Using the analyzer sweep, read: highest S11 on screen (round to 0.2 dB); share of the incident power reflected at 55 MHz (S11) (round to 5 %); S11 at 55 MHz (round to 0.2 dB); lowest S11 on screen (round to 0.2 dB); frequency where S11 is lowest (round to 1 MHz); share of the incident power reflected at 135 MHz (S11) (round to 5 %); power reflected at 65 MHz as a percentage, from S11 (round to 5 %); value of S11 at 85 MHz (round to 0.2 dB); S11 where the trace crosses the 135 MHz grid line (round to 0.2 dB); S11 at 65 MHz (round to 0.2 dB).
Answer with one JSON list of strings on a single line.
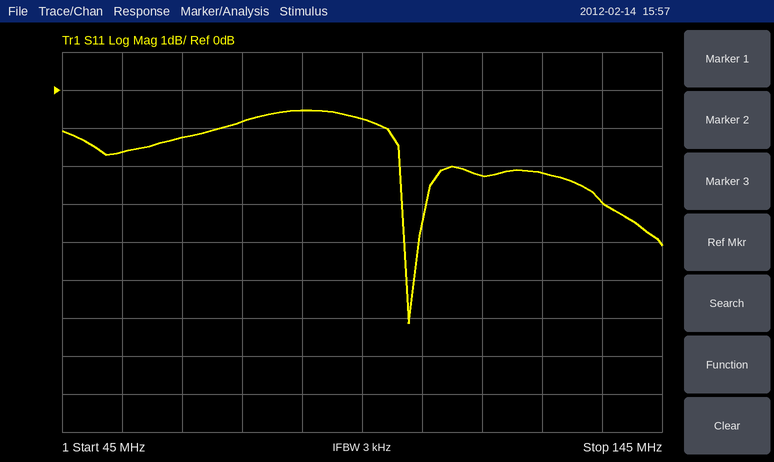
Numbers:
["-0.6 dB", "70 %", "-1.6 dB", "-6.2 dB", "103 MHz", "50 %", "75 %", "-0.6 dB", "-3.0 dB", "-1.2 dB"]
